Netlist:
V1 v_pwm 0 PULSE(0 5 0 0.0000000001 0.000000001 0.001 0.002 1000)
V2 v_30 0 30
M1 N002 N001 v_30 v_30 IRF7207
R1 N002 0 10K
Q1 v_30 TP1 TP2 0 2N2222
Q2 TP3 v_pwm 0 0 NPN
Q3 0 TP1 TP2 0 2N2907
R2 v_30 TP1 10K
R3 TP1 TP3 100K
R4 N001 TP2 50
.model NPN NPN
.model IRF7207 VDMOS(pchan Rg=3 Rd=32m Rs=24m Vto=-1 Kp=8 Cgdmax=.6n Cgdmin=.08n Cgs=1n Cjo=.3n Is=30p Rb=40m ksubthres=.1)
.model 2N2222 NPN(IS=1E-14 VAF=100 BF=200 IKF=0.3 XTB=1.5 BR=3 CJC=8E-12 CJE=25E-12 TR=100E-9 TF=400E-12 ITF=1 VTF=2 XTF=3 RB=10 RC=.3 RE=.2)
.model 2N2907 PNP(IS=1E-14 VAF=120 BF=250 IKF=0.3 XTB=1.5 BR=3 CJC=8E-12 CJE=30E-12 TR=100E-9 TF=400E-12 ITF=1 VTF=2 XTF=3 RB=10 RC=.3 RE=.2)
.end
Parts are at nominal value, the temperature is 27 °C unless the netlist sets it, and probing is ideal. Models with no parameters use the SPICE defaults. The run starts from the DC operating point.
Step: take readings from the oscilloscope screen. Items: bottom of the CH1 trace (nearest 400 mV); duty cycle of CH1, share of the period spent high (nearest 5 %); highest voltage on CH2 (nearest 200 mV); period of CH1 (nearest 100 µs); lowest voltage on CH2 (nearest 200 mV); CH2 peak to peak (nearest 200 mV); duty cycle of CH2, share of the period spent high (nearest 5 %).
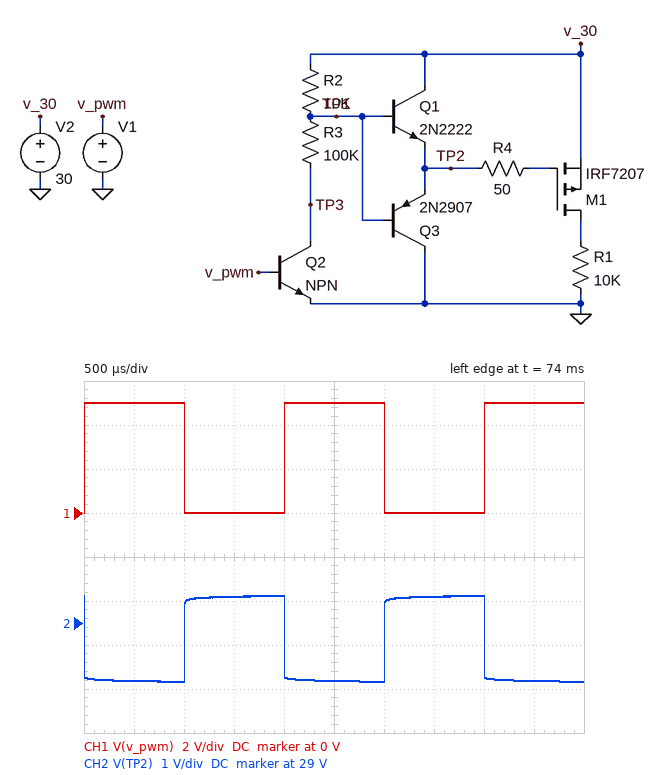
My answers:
0 V
50 %
29.6 V
2.0 ms
27.6 V
2.0 V
50 %
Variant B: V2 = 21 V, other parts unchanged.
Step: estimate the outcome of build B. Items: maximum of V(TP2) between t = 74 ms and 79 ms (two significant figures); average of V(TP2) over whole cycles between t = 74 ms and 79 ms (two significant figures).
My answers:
21 V
20 V
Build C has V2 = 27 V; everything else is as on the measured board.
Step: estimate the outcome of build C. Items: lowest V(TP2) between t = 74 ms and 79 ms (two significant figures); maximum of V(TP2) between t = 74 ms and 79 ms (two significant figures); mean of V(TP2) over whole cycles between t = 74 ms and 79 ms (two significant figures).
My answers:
25 V
27 V
26 V
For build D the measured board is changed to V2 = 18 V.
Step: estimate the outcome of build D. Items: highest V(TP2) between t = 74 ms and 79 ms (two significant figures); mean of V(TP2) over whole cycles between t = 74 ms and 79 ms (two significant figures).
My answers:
18 V
17 V
